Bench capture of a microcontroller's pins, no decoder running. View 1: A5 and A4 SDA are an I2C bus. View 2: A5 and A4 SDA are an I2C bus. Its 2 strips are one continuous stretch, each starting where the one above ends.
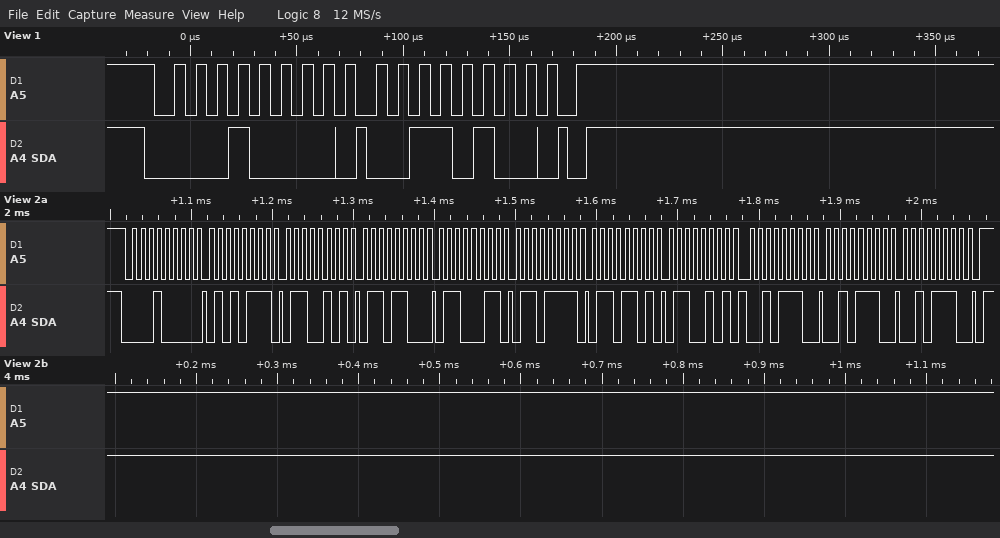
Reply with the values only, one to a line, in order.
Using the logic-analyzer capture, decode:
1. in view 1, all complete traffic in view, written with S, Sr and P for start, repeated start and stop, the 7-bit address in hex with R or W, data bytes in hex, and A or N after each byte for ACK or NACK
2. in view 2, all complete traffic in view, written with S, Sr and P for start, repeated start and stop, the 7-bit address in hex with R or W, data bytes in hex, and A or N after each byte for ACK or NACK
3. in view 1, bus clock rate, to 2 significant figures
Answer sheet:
S 08W A 34 A P
S 08W A 57 A 65 A 6C A 63 A 6F A 6D A 65 A 2E A 2E A 2E A P
100 kHz
